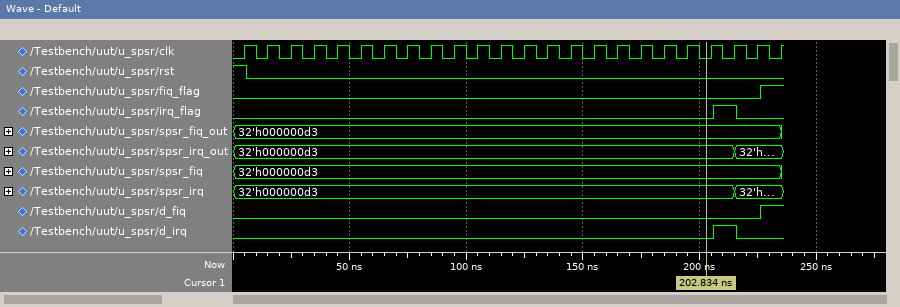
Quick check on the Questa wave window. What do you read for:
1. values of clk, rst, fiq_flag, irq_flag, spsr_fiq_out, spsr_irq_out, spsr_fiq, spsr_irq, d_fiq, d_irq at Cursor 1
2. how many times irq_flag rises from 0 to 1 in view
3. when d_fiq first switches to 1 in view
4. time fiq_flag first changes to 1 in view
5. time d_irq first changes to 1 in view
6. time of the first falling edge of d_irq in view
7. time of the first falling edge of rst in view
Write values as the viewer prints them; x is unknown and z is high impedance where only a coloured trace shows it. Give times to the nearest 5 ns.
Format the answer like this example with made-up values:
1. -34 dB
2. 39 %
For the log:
1. clk=0, rst=0, fiq_flag=0, irq_flag=0, spsr_fiq_out=32'h000000d3, spsr_irq_out=32'h000000d3, spsr_fiq=32'h000000d3, spsr_irq=32'h000000d3, d_fiq=0, d_irq=0
2. 1
3. 225 ns
4. 225 ns
5. 205 ns
6. 215 ns
7. 5 ns
